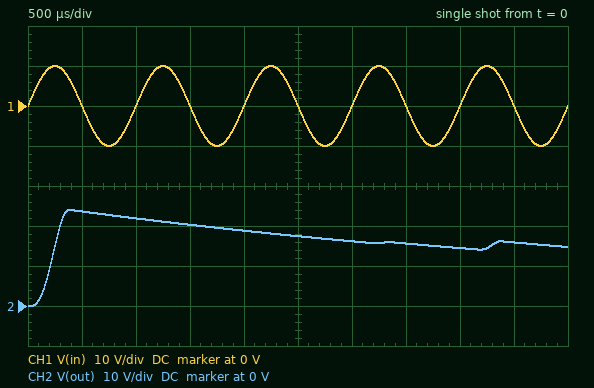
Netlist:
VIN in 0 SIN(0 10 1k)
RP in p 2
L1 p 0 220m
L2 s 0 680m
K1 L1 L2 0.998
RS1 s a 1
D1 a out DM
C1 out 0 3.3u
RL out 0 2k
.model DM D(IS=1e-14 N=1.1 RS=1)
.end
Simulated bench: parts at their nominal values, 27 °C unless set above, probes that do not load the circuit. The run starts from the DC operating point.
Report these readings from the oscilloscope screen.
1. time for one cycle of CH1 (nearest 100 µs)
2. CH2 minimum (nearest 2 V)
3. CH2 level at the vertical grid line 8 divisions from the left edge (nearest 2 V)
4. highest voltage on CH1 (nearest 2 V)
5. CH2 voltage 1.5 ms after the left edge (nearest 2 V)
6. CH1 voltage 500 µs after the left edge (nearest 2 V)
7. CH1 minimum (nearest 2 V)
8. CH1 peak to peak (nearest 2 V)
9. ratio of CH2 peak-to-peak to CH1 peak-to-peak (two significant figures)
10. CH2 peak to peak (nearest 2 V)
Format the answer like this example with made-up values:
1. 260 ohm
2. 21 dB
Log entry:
1. 1.0 ms
2. 0 V
3. 14 V
4. 10 V
5. 20 V
6. 0 V
7. -10 V
8. 20 V
9. 1.2
10. 24 V
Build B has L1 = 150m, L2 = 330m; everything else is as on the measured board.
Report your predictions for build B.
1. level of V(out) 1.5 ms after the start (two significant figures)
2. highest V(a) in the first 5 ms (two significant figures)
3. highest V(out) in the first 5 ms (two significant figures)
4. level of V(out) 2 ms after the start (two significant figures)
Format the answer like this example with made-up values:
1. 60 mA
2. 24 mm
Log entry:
1. 16 V
2. 20 V
3. 19 V
4. 15 V
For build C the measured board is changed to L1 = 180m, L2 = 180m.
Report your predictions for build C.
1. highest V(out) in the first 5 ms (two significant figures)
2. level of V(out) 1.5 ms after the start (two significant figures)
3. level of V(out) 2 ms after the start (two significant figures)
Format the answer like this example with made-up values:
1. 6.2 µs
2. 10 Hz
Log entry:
1. 12 V
2. 9.7 V
3. 9.0 V
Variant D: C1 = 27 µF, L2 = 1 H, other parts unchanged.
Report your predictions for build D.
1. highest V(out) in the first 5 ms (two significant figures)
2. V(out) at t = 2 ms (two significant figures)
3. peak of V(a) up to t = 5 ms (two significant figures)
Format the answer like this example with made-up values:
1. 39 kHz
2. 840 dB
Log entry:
1. 16 V
2. 13 V
3. 17 V
